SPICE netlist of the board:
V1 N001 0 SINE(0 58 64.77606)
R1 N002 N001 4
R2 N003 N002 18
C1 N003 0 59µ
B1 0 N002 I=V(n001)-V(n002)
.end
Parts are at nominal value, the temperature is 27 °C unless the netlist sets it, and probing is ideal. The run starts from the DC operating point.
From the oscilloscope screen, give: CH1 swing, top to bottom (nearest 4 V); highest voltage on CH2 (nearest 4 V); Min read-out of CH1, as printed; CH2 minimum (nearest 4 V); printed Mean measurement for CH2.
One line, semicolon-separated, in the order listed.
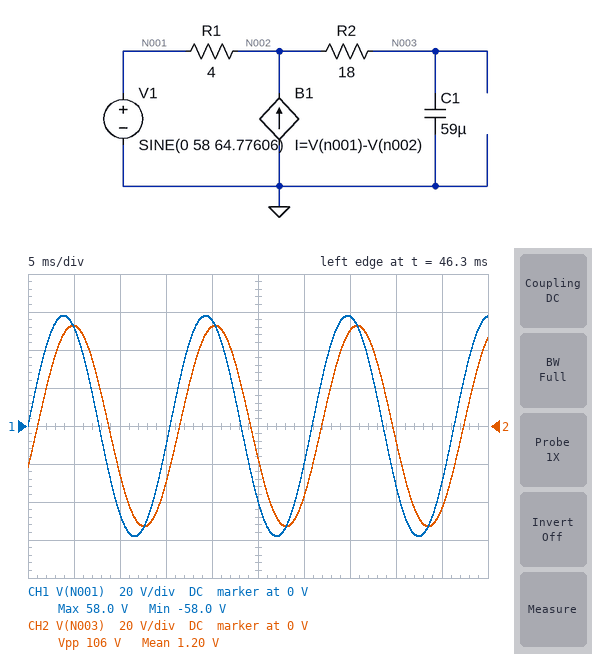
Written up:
116 V; 52 V; -58.0 V; -52 V; 1.20 V
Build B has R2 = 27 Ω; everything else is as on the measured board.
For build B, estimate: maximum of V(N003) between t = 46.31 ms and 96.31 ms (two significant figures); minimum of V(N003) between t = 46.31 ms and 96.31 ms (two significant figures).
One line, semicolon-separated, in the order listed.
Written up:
48 V; -48 V
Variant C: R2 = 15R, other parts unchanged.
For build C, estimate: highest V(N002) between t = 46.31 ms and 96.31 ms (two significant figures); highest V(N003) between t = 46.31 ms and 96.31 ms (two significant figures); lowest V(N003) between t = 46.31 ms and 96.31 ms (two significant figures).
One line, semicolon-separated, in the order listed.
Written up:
58 V; 54 V; -54 V
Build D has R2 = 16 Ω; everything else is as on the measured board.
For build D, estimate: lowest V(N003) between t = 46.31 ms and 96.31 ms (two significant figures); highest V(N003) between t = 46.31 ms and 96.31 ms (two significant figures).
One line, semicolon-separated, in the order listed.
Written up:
-54 V; 54 V
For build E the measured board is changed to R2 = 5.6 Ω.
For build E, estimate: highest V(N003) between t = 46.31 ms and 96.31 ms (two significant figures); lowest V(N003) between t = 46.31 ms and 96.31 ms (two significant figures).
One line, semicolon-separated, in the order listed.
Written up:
57 V; -57 V
